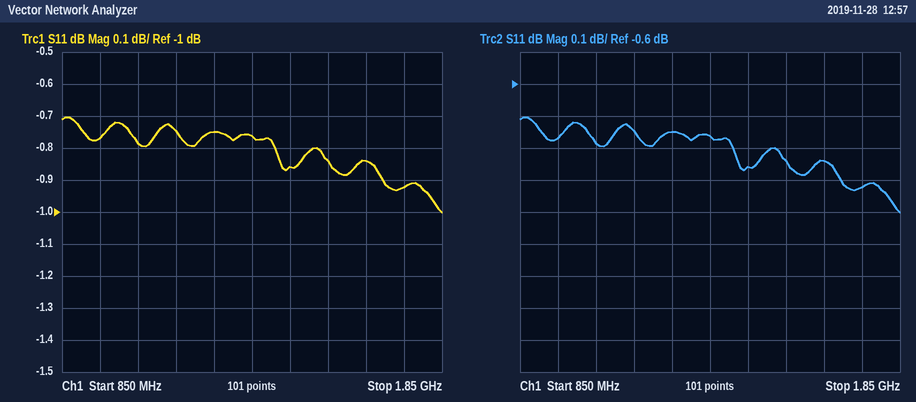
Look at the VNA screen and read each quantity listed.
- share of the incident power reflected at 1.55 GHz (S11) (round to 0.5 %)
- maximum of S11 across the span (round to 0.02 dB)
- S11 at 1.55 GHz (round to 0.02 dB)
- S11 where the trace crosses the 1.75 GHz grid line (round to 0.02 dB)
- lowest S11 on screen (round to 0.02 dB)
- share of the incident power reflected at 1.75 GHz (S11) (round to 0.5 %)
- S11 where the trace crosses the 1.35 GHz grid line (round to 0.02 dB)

82.5 %
-0.70 dB
-0.84 dB
-0.92 dB
-1.00 dB
81.0 %
-0.76 dB
